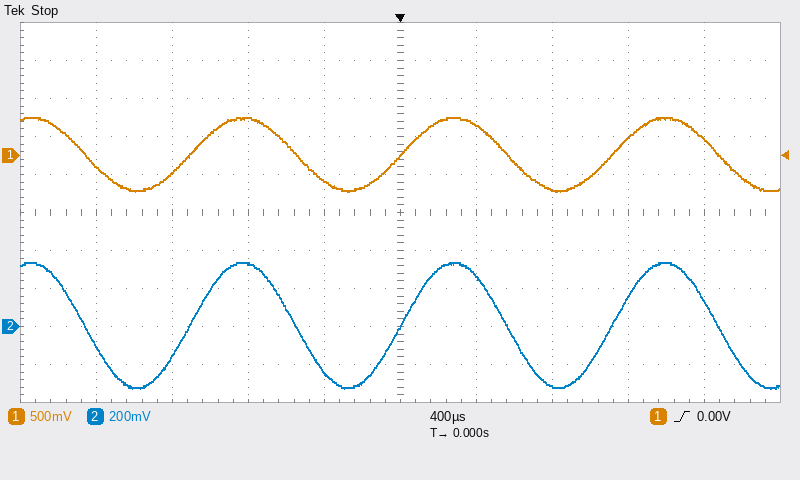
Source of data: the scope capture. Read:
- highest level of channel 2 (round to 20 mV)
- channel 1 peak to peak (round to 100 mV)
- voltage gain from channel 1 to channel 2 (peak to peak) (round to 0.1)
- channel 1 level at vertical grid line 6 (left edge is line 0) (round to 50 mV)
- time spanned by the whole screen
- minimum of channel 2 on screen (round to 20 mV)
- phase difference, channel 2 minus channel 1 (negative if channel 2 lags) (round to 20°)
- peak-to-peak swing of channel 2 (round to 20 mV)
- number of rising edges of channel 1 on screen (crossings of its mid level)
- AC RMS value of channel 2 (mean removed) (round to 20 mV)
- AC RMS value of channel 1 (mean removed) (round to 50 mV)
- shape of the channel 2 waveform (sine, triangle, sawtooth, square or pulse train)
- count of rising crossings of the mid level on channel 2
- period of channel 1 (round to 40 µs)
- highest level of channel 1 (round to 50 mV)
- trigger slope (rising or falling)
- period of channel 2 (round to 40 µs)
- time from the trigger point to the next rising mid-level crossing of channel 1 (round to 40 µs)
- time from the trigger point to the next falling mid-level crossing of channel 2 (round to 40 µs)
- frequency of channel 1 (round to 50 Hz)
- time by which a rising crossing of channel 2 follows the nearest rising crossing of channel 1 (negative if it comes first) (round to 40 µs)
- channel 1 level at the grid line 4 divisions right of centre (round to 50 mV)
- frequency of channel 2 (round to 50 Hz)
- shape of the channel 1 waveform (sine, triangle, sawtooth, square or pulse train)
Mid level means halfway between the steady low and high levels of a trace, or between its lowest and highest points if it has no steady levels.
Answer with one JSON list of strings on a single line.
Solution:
["340 mV", "1.00 V", "0.7", "400 mV", "4 ms", "-320 mV", "0°", "660 mV", "3", "240 mV", "350 mV", "sine", "3", "1.12 ms", "500 mV", "rising", "1.12 ms", "1.12 ms", "560 µs", "900 Hz", "0 µs", "200 mV", "900 Hz", "sine"]
